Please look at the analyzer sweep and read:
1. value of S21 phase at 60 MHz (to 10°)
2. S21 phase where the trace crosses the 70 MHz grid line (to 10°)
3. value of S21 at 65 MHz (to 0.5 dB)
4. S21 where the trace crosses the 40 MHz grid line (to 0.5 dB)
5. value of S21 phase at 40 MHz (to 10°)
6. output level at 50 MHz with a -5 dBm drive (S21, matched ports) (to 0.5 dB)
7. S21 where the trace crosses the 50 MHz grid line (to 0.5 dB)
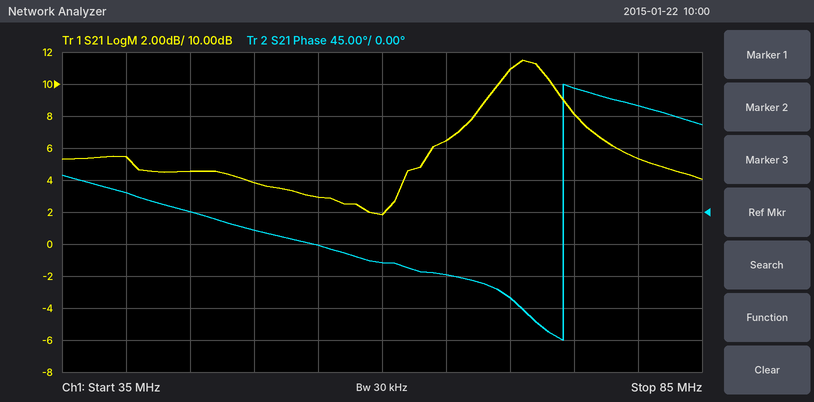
-70°
-120°
6.5 dB
5.5 dB
30°
-1.0 dBm
4.0 dB
